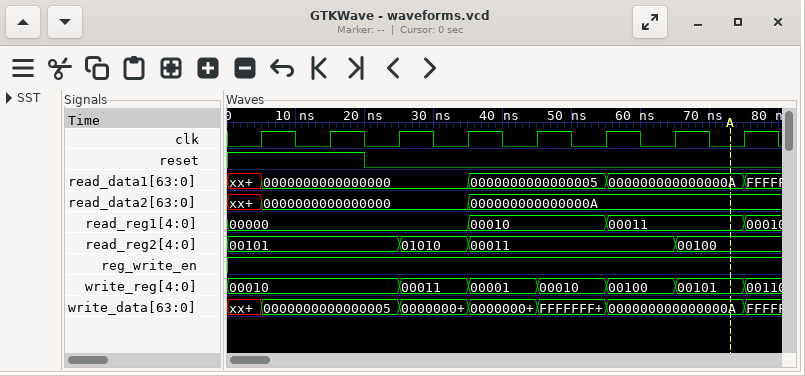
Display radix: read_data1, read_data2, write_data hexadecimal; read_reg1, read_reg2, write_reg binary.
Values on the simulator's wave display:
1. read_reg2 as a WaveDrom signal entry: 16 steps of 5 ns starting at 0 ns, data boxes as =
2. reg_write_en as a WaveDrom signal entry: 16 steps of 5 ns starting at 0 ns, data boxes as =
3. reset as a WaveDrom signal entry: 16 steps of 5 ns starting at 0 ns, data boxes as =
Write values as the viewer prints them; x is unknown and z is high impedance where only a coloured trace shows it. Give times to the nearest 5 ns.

{name: 'read_reg2', wave: '=....=.=.....=..', data: '00101 01010 00011 00100'}
{name: 'reg_write_en', wave: '1...............'}
{name: 'reset', wave: '1...0...........'}
